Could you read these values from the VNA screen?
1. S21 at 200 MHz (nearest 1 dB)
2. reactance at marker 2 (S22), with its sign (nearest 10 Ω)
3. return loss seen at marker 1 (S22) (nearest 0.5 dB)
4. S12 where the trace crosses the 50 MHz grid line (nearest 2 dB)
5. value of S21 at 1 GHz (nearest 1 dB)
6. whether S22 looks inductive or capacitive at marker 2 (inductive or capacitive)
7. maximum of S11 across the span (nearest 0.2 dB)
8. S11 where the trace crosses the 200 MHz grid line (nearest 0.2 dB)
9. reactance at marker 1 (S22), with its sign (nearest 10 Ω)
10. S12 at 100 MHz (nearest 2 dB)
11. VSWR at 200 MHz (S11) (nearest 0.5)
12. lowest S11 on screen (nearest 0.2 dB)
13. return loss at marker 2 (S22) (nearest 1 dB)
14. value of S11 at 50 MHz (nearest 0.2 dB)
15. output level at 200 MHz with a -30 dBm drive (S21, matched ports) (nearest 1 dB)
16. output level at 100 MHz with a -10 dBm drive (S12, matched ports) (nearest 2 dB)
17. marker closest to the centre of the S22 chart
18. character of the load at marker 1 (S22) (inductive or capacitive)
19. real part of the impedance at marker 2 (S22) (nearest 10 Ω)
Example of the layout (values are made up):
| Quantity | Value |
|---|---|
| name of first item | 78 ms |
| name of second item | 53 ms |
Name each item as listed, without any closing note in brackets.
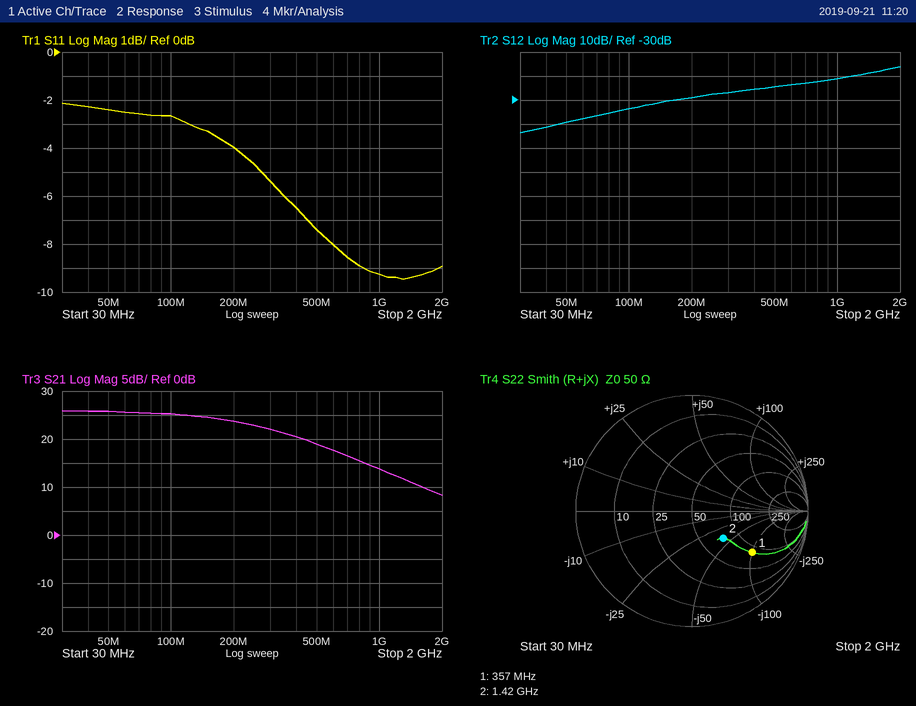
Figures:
| Quantity | Value |
|---|---|
| S21 at 200 MHz | 24 dB |
| reactance at marker 2 (S22), with its sign | -40 Ω |
| return loss seen at marker 1 (S22) | 4.0 dB |
| S12 where the trace crosses the 50 MHz grid line | -40 dB |
| value of S21 at 1 GHz | 14 dB |
| whether S22 looks inductive or capacitive at marker 2 | capacitive |
| maximum of S11 across the span | -2.2 dB |
| S11 where the trace crosses the 200 MHz grid line | -4.0 dB |
| reactance at marker 1 (S22), with its sign | -100 Ω |
| S12 at 100 MHz | -34 dB |
| VSWR at 200 MHz (S11) | 4.5 |
| lowest S11 on screen | -9.4 dB |
| return loss at marker 2 (S22) | 9 dB |
| value of S11 at 50 MHz | -2.4 dB |
| output level at 200 MHz with a -30 dBm drive (S21, matched ports) | -6 dBm |
| output level at 100 MHz with a -10 dBm drive (S12, matched ports) | -44 dBm |
| marker closest to the centre of the S22 chart | marker 2 |
| character of the load at marker 1 (S22) | capacitive |
| real part of the impedance at marker 2 (S22) | 70 Ω |
